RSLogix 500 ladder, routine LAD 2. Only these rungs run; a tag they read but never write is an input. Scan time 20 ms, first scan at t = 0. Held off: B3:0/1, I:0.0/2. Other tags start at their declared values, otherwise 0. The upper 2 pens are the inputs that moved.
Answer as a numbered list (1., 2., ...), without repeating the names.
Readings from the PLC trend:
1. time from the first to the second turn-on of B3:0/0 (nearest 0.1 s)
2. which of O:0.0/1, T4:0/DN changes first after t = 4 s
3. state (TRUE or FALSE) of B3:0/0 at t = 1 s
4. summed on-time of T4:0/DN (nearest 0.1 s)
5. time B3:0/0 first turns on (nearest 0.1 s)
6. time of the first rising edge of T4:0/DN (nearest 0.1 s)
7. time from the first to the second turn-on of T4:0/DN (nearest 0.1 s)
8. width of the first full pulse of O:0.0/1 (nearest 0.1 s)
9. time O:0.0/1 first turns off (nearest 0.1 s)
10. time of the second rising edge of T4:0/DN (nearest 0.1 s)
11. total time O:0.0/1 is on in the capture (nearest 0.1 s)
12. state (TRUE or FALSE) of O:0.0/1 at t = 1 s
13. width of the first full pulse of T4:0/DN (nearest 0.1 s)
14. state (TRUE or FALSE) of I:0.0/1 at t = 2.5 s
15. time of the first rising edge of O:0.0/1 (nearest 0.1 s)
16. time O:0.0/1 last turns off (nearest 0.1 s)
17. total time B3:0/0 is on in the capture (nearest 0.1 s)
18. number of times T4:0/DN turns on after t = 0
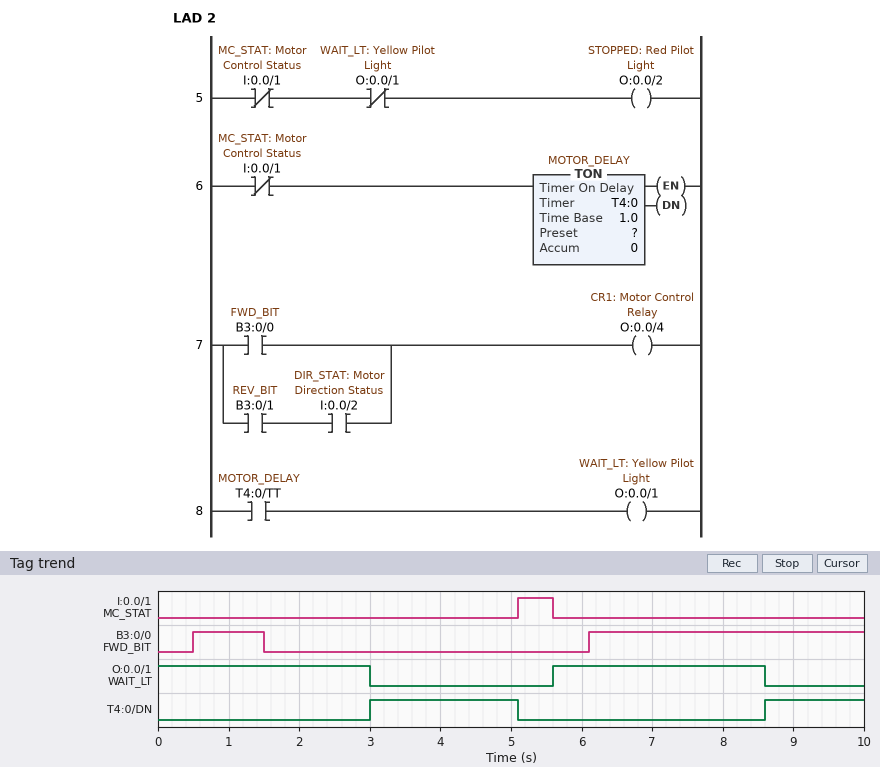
1. 5.6 s
2. T4:0/DN
3. TRUE
4. 3.5 s
5. 0.5 s
6. 3.0 s
7. 5.6 s
8. 3.0 s
9. 3.0 s
10. 8.6 s
11. 6.0 s
12. TRUE
13. 2.1 s
14. FALSE
15. 5.6 s
16. 8.6 s
17. 4.9 s
18. 2
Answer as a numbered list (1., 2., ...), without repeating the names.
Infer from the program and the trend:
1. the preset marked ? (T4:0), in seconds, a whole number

1. 3 s
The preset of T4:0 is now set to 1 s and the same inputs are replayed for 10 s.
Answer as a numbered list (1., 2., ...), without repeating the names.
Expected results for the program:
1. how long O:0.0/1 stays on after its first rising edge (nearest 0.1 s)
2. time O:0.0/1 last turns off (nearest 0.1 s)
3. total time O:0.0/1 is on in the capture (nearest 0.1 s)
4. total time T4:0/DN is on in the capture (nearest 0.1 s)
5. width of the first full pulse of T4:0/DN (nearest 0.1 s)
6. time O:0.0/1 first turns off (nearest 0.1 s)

1. 1.0 s
2. 6.6 s
3. 2.0 s
4. 7.5 s
5. 4.1 s
6. 1.0 s
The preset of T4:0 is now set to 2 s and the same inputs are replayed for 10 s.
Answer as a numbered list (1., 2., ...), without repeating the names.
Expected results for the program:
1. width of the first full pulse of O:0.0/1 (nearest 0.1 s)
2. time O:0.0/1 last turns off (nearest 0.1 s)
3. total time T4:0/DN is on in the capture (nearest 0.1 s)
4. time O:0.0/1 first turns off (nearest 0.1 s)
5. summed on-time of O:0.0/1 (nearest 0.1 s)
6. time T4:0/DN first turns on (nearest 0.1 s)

1. 2.0 s
2. 7.6 s
3. 5.5 s
4. 2.0 s
5. 4.0 s
6. 2.0 s
